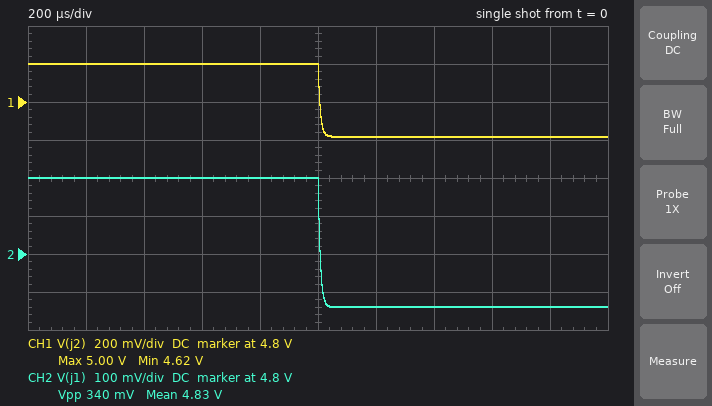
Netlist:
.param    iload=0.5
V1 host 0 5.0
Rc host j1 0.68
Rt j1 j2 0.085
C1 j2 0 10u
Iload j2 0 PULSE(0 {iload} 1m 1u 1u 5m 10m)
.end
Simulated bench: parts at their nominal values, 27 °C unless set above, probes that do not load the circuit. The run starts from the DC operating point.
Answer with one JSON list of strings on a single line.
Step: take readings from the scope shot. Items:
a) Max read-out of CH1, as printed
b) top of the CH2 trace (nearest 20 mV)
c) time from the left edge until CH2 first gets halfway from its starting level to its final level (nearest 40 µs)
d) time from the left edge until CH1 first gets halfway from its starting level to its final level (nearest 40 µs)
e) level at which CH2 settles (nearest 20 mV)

["5.00 V", "5.00 V", "1.00 ms", "1.00 ms", "4.66 V"]
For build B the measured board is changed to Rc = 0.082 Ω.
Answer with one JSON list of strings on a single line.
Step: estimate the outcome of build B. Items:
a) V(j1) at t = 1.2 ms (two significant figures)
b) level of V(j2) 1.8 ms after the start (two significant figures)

["5.0 V", "4.9 V"]
